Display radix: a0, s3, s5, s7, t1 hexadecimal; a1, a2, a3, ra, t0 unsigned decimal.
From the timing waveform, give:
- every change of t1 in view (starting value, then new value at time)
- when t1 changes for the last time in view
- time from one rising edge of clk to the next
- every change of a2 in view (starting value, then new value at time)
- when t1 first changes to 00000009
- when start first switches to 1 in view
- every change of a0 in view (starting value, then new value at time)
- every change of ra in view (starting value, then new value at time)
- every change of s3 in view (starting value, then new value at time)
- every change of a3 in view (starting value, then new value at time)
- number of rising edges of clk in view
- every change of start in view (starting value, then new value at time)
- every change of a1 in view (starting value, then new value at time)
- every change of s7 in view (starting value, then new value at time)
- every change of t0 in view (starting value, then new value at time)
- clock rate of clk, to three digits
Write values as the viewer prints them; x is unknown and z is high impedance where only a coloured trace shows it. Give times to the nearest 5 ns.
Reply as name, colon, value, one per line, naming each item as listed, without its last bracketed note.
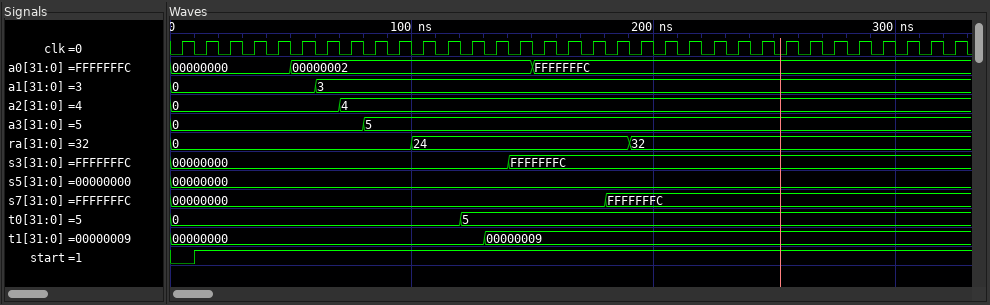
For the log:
every change of t1 in view: 00000000, 00000009 at 130 ns
when t1 changes for the last time in view: 130 ns
time from one rising edge of clk to the next: 10 ns
every change of a2 in view: 0, 4 at 70 ns
when t1 first changes to 00000009: 130 ns
when start first switches to 1 in view: 10 ns
every change of a0 in view: 00000000, 00000002 at 50 ns, FFFFFFFC at 150 ns
every change of ra in view: 0, 24 at 100 ns, 32 at 190 ns
every change of s3 in view: 00000000, FFFFFFFC at 140 ns
every change of a3 in view: 0, 5 at 80 ns
number of rising edges of clk in view: 33
every change of start in view: 0, 1 at 10 ns
every change of a1 in view: 0, 3 at 60 ns
every change of s7 in view: 00000000, FFFFFFFC at 180 ns
every change of t0 in view: 0, 5 at 120 ns
clock rate of clk, to three digits: 100 MHz
